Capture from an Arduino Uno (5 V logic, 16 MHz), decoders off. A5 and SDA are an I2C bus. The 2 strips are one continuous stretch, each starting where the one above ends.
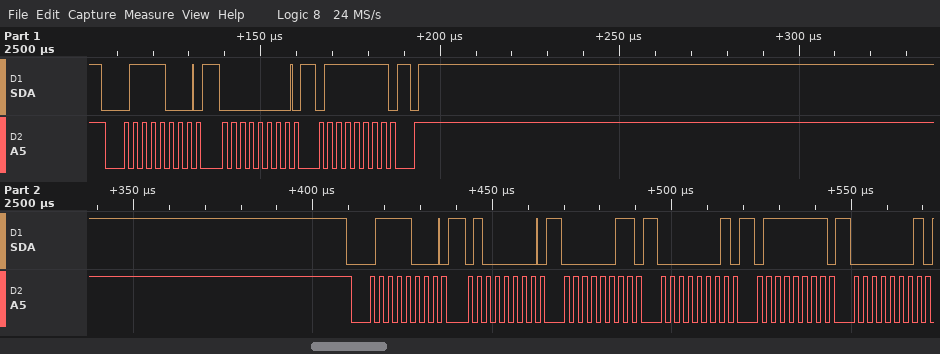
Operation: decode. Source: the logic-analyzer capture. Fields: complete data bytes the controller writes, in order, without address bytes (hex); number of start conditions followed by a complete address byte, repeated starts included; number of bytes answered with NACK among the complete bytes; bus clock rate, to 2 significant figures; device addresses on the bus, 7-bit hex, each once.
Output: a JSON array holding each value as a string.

["00 7F 40 03 01 7F 01", "2", "0", "400 kHz", "0x3C"]
